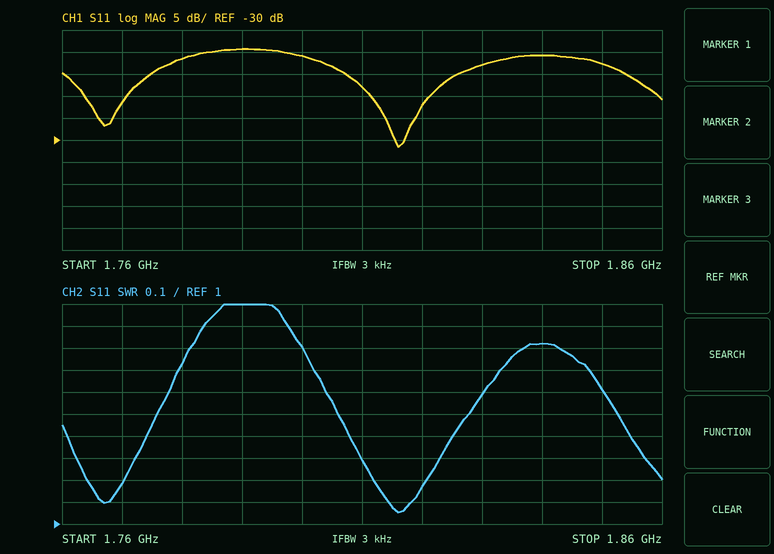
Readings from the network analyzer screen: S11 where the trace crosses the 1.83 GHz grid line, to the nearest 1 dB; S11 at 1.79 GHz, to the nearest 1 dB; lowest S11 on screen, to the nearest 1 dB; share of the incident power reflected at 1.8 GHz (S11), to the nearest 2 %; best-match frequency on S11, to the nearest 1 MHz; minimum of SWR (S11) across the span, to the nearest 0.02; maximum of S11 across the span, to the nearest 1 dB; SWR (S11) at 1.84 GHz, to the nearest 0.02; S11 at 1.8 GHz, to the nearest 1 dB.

-13 dB
-9 dB
-32 dB
8 %
1.816 GHz
1.06
-9 dB
1.82
-11 dB
